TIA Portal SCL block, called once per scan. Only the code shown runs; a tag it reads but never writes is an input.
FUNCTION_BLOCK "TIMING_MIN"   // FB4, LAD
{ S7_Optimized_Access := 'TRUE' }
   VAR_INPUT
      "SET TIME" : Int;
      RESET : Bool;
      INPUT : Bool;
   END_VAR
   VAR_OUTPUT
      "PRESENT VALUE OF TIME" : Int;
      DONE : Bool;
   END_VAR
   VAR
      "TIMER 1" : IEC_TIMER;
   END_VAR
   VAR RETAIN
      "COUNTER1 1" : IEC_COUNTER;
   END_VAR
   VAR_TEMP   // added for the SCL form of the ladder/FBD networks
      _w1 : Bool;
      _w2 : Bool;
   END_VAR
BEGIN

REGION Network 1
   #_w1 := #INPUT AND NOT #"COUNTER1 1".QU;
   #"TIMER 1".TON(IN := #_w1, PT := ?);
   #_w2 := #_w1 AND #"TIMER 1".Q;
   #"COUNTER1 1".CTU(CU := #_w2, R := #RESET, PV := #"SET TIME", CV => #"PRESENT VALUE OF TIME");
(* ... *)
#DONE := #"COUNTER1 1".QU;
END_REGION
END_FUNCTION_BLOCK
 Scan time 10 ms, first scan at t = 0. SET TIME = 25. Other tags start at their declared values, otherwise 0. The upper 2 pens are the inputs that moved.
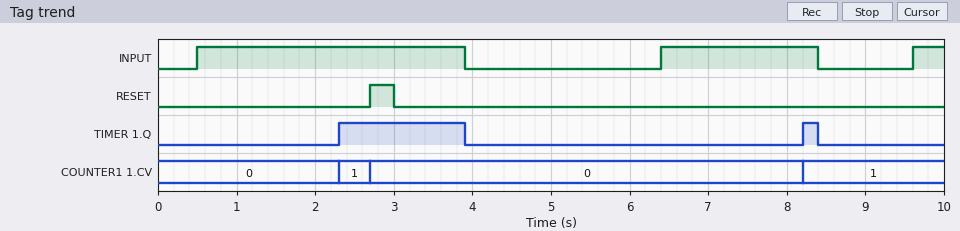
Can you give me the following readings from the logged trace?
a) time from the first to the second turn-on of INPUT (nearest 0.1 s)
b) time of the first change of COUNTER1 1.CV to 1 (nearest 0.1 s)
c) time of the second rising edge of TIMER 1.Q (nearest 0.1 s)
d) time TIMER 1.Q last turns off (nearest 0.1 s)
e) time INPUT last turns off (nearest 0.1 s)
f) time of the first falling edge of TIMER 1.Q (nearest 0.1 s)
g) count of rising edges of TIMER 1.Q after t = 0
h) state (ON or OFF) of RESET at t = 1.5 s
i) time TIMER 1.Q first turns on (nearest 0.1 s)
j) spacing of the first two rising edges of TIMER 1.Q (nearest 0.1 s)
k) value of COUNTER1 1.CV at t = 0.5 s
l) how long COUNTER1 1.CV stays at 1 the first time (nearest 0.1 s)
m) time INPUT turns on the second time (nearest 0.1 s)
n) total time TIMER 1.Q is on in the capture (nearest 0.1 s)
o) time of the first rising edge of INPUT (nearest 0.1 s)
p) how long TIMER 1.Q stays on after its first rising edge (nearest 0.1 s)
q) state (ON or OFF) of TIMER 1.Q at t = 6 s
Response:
5.9 s
2.3 s
8.2 s
8.4 s
8.4 s
3.9 s
2
OFF
2.3 s
5.9 s
0
0.4 s
6.4 s
1.8 s
0.5 s
1.6 s
OFF
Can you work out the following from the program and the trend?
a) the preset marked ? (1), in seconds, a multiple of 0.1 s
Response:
1.8 s
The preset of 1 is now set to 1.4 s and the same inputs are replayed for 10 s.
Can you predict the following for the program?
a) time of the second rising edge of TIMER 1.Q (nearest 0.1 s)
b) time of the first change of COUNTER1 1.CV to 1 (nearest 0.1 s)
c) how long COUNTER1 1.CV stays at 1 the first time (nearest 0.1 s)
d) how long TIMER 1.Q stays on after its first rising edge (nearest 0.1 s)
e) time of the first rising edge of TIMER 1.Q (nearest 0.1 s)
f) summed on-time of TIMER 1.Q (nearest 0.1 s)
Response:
7.8 s
1.9 s
0.8 s
2.0 s
1.9 s
2.6 s
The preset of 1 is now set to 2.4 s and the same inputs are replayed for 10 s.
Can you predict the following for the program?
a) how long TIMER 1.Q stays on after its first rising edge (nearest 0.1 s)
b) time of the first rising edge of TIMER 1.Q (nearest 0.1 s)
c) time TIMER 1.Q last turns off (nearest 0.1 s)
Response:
1.0 s
2.9 s
3.9 s
